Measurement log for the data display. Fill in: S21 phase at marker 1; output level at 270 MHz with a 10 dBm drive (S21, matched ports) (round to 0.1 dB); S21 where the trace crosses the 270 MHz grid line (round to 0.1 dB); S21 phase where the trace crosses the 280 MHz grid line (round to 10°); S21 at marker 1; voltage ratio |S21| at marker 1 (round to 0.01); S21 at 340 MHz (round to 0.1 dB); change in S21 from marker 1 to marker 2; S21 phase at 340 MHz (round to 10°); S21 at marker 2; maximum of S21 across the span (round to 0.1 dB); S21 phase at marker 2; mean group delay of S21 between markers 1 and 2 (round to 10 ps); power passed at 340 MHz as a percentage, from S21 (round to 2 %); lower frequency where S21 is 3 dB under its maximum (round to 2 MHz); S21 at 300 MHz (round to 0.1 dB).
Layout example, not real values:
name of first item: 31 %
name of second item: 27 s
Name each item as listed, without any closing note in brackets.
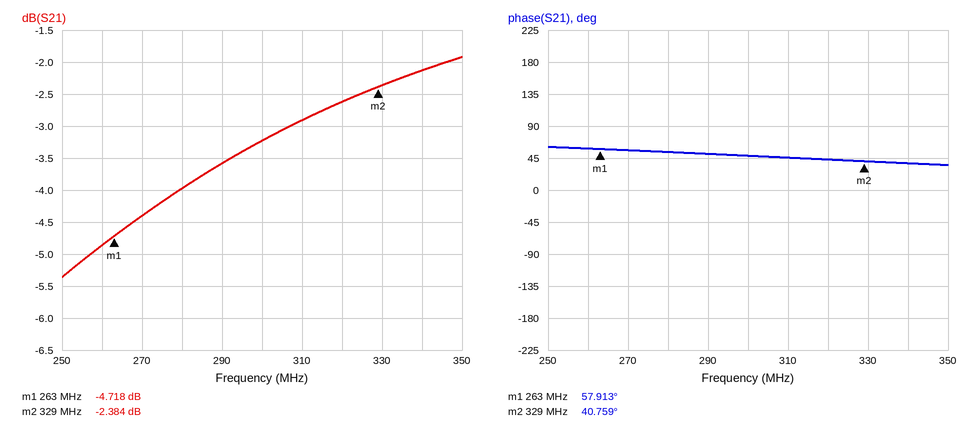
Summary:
S21 phase at marker 1: 57.913°
output level at 270 MHz with a 10 dBm drive (S21, matched ports): 5.6 dBm
S21 where the trace crosses the 270 MHz grid line: -4.4 dB
S21 phase where the trace crosses the 280 MHz grid line: 50°
S21 at marker 1: -4.718 dB
voltage ratio |S21| at marker 1: 0.58
S21 at 340 MHz: -2.1 dB
change in S21 from marker 1 to marker 2: 2.334 dB
S21 phase at 340 MHz: 40°
S21 at marker 2: -2.384 dB
maximum of S21 across the span: -1.9 dB
S21 phase at marker 2: 40.759°
mean group delay of S21 between markers 1 and 2: 720 ps
power passed at 340 MHz as a percentage, from S21: 62 %
lower frequency where S21 is 3 dB under its maximum: 258 MHz
S21 at 300 MHz: -3.2 dB
